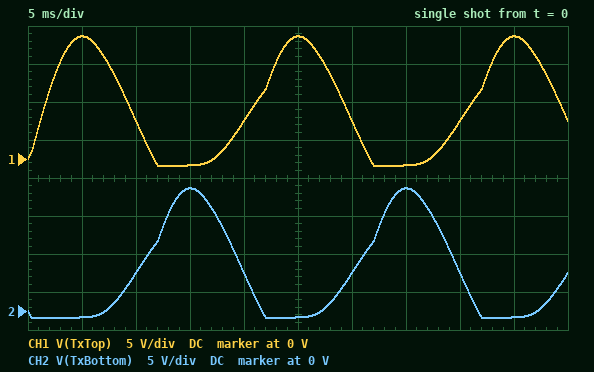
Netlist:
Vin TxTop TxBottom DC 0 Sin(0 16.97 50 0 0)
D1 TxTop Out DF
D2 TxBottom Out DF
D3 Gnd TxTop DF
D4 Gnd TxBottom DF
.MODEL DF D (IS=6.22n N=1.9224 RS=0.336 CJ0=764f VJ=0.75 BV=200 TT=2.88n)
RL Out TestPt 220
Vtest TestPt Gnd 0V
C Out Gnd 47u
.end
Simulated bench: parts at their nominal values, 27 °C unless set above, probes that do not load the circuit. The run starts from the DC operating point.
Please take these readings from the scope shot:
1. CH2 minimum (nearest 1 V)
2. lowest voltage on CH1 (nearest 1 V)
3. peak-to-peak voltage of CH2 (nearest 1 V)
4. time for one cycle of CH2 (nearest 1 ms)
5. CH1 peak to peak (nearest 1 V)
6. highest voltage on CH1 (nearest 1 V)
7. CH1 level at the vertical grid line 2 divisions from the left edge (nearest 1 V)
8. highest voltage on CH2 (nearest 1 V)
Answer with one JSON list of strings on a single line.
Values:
["-1 V", "-1 V", "17 V", "20 ms", "17 V", "16 V", "5 V", "16 V"]
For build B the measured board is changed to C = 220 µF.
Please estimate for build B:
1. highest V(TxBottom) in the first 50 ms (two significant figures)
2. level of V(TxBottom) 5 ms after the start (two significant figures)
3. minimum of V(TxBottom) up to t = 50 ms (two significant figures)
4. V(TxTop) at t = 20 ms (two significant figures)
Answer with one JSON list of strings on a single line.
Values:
["16 V", "-900 mV", "-1.3 V", "6.9 V"]
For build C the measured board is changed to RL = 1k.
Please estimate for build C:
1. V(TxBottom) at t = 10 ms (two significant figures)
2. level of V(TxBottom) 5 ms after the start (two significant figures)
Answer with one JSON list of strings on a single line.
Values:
["7.0 V", "-770 mV"]
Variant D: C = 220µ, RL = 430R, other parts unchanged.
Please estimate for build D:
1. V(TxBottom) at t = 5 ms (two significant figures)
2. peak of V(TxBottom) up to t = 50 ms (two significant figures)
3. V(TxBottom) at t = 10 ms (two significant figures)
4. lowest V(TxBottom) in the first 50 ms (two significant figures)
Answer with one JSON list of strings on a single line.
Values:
["-880 mV", "16 V", "7.3 V", "-1.3 V"]
